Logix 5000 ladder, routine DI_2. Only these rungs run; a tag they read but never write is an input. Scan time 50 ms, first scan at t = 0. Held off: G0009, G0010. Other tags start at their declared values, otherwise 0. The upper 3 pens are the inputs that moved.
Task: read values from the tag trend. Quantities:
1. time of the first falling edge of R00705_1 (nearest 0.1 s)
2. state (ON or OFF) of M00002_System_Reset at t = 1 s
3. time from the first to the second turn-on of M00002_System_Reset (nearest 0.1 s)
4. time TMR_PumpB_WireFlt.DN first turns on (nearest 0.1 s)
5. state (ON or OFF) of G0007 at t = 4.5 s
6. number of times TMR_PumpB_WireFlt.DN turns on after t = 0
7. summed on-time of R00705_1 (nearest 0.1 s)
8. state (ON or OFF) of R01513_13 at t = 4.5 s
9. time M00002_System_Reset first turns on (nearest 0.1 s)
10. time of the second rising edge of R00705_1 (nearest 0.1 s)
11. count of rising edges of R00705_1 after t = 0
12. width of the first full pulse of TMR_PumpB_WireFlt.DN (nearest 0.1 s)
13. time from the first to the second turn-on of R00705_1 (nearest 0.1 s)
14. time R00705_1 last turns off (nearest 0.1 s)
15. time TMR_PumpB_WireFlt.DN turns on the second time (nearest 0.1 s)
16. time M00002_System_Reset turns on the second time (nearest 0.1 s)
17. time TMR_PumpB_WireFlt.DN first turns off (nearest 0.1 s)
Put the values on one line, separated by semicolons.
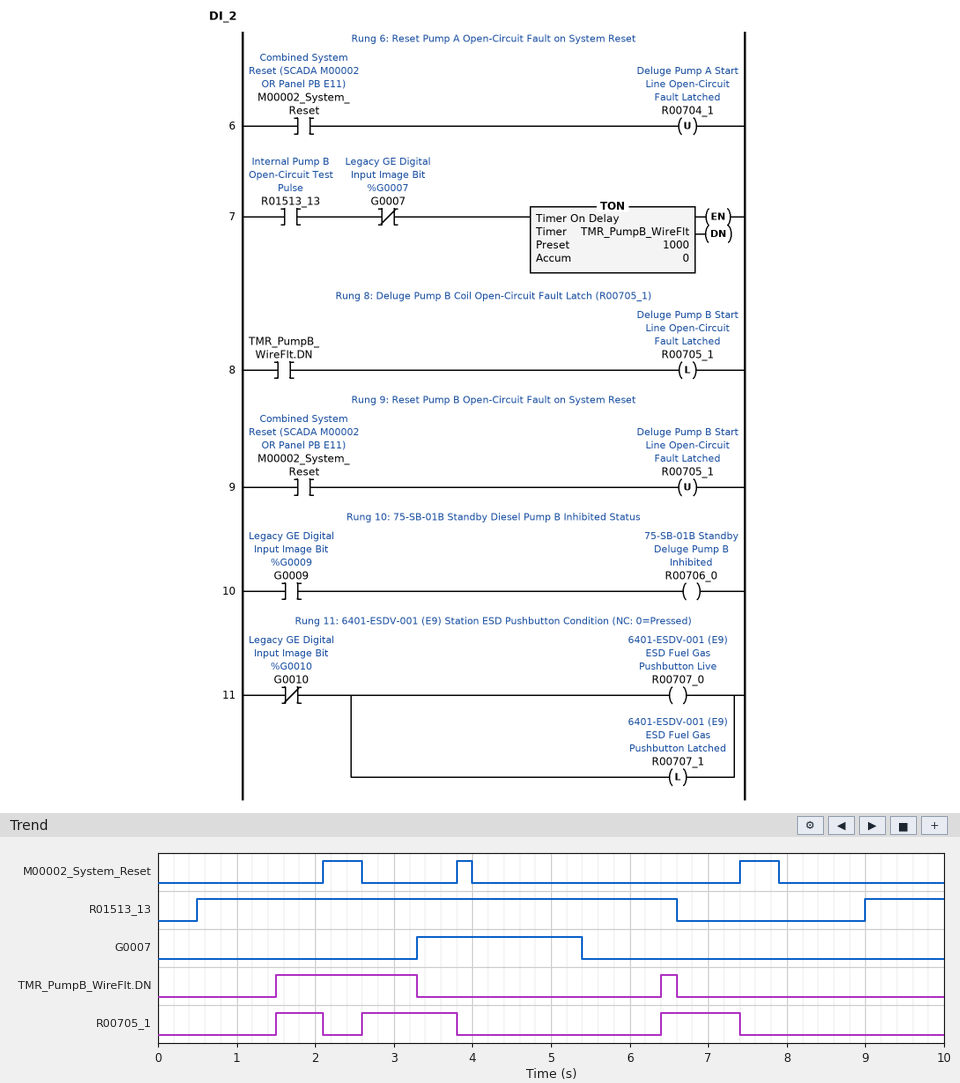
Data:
2.1 s; OFF; 1.7 s; 1.5 s; ON; 2; 2.8 s; ON; 2.1 s; 2.6 s; 3; 1.8 s; 1.1 s; 7.4 s; 6.4 s; 3.8 s; 3.3 s
